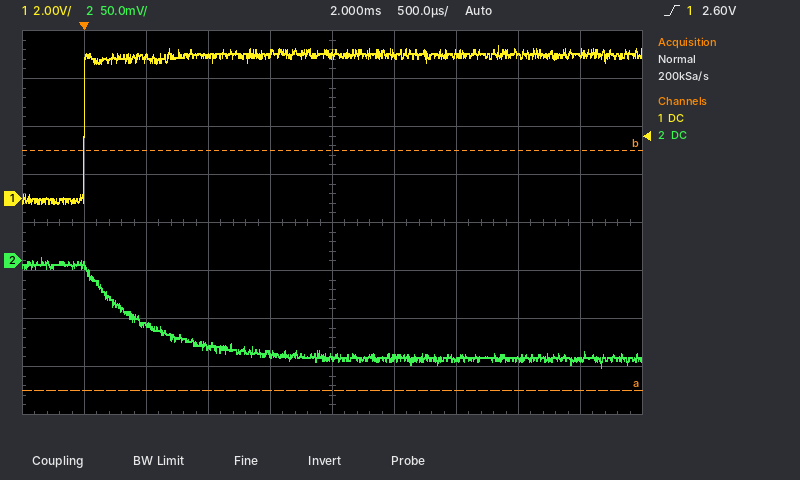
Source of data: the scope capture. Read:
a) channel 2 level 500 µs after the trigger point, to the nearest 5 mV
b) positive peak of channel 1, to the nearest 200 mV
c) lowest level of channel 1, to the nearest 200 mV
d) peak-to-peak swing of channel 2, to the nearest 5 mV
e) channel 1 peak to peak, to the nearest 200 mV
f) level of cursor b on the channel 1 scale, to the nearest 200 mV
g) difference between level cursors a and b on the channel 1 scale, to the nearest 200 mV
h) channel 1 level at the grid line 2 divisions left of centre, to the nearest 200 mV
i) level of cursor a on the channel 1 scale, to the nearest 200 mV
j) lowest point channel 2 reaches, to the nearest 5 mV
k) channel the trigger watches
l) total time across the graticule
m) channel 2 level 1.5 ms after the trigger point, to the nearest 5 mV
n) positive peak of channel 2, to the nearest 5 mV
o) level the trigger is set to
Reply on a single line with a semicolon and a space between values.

-65 mV; 6.4 V; -200 mV; 115 mV; 6.6 V; 2.0 V; 10.0 V; 6.0 V; -8.0 V; -110 mV; channel 1; 5 ms; -95 mV; 5 mV; 2.60 V
